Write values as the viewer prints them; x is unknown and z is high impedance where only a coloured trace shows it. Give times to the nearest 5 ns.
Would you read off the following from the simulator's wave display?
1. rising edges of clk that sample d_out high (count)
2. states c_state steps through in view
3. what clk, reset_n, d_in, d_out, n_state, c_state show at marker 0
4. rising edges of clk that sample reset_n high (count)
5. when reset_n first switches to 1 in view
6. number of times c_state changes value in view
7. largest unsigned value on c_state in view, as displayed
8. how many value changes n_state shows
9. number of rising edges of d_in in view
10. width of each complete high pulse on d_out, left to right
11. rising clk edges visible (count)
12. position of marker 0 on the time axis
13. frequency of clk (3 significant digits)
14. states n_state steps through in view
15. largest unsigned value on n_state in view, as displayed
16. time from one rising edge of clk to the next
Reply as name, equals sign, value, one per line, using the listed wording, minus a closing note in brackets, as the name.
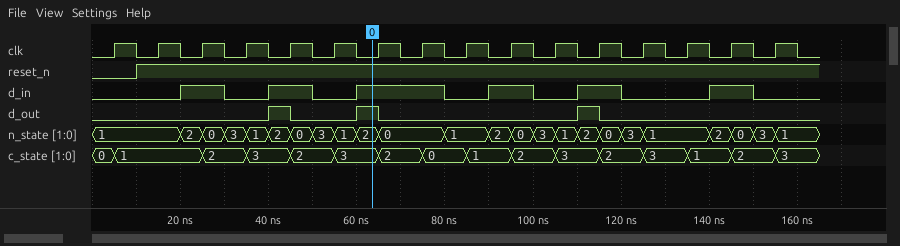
rising edges of clk that sample d_out high = 3
states c_state steps through in view = 0, 1, 2, 3, 2, 3, 2, 0, 1, 2, 3, 2, 3, 1, 2, 3
what clk, reset_n, d_in, d_out, n_state, c_state show at marker 0 = clk=0, reset_n=1, d_in=1, d_out=1, n_state=2, c_state=3
rising edges of clk that sample reset_n high = 15
when reset_n first switches to 1 in view = 10 ns
number of times c_state changes value in view = 15
largest unsigned value on c_state in view, as displayed = 3
how many value changes n_state shows = 23
number of rising edges of d_in in view = 6
width of each complete high pulse on d_out, left to right = 5 ns, 5 ns, 5 ns
rising clk edges visible = 16
position of marker 0 on the time axis = 65 ns
frequency of clk = 100 MHz
states n_state steps through in view = 1, 2, 0, 3, 1, 2, 0, 3, 1, 2, 0, 1, 2, 0, 3, 1, 2, 0, 3, 1, 2, 0, 3, 1
largest unsigned value on n_state in view, as displayed = 3
time from one rising edge of clk to the next = 10 ns
